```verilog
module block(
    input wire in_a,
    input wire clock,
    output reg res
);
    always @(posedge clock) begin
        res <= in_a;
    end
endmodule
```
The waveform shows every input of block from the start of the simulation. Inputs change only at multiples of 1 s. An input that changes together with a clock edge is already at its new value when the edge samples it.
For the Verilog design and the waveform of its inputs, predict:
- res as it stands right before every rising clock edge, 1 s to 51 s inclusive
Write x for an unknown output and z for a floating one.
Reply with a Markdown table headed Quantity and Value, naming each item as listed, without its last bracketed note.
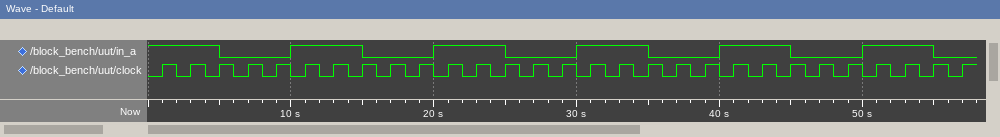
| Quantity | Value |
|---|---|
| res as it stands right before every rising clock edge, 1 s to 51 s inclusive | x 1 1 0 0 0 1 1 0 0 0 1 1 0 0 0 1 1 0 0 0 1 1 0 0 0 |
